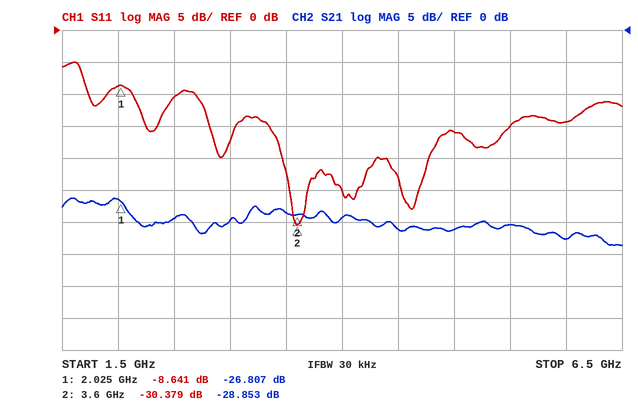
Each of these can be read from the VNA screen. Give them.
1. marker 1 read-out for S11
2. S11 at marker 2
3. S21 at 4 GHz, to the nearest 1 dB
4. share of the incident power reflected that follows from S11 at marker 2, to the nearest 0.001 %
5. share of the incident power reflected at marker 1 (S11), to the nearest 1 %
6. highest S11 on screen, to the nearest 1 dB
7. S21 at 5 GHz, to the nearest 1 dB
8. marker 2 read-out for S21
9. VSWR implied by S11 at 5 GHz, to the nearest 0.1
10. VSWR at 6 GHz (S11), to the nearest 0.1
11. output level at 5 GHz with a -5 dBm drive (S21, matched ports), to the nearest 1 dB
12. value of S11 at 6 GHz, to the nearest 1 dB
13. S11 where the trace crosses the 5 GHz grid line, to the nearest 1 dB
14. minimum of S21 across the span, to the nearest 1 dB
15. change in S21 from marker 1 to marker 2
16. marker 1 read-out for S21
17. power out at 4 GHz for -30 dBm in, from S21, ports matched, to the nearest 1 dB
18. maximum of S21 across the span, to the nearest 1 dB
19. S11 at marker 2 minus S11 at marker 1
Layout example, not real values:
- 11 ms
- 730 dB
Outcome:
- -8.641 dB
- -30.379 dB
- -29 dB
- 0.092 %
- 14 %
- -5 dB
- -31 dB
- -28.853 dB
- 1.4
- 1.5
- -36 dBm
- -14 dB
- -16 dB
- -34 dB
- -2.046 dB
- -26.807 dB
- -59 dBm
- -26 dB
- -21.738 dB
